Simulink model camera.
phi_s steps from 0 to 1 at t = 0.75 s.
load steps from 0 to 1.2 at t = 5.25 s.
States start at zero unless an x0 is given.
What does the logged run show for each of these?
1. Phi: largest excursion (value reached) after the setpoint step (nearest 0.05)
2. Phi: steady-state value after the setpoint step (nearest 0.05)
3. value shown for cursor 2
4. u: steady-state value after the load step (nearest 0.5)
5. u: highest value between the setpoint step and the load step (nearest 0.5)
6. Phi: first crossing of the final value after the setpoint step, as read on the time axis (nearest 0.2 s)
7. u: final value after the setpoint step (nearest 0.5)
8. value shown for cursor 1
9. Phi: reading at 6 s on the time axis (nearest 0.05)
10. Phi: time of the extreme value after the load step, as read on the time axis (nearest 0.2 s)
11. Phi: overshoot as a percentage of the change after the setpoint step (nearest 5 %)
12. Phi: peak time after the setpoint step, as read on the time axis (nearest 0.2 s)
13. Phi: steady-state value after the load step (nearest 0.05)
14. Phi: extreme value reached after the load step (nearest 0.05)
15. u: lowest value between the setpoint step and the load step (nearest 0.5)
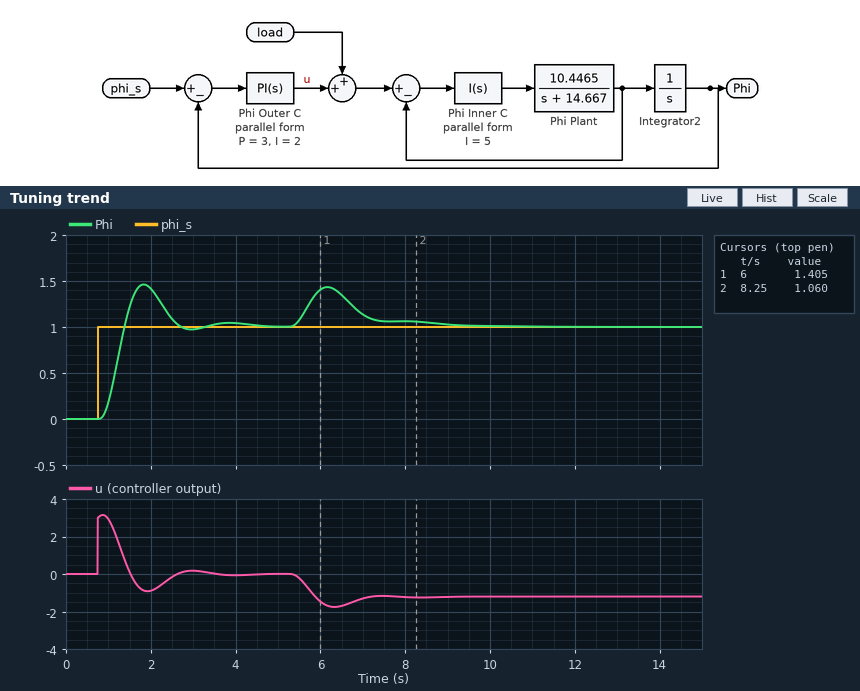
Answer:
1.45
1.00
1.060
-1.0
3.0
1.4 s
0.0
1.405
1.40
6.2 s
45 %
1.8 s
1.00
1.45
-1.0
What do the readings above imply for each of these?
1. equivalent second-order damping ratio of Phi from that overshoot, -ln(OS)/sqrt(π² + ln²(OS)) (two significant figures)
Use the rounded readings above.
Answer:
0.25
